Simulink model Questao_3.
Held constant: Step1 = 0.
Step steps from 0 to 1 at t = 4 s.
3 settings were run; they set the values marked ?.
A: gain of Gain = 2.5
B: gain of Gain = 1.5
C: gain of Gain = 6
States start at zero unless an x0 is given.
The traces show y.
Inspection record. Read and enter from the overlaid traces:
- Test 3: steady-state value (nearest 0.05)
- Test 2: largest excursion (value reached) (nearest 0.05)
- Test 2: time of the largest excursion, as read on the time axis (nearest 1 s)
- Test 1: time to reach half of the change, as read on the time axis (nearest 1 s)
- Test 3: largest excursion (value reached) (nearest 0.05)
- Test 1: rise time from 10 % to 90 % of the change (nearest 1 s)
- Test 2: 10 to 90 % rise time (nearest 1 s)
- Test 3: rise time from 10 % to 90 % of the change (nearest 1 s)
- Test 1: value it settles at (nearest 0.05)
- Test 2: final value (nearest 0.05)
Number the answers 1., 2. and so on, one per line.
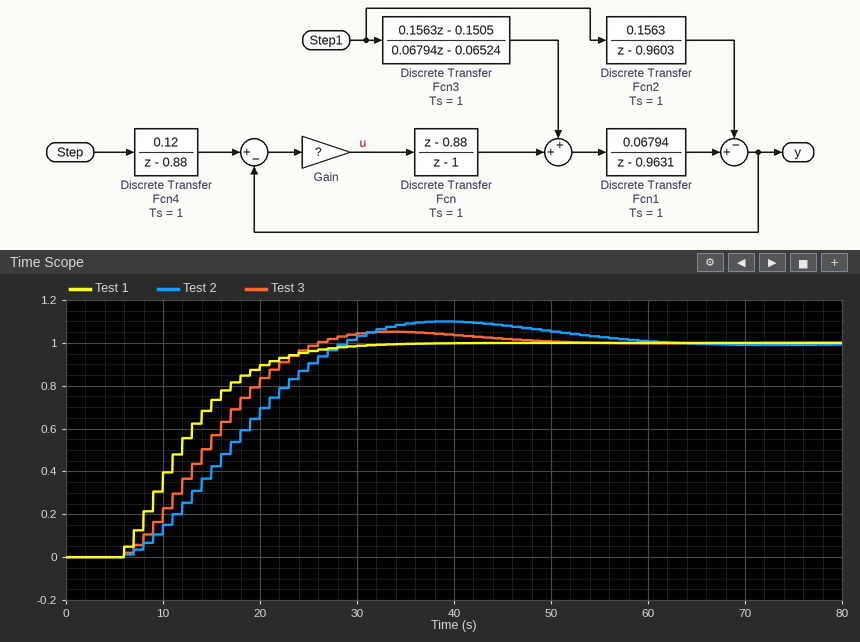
1. 1.00
2. 1.10
3. 39 s
4. 12 s
5. 1.05
6. 14 s
7. 16 s
8. 14 s
9. 1.00
10. 1.00
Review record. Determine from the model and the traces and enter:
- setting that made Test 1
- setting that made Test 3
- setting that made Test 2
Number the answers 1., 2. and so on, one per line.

1. C
2. A
3. B
